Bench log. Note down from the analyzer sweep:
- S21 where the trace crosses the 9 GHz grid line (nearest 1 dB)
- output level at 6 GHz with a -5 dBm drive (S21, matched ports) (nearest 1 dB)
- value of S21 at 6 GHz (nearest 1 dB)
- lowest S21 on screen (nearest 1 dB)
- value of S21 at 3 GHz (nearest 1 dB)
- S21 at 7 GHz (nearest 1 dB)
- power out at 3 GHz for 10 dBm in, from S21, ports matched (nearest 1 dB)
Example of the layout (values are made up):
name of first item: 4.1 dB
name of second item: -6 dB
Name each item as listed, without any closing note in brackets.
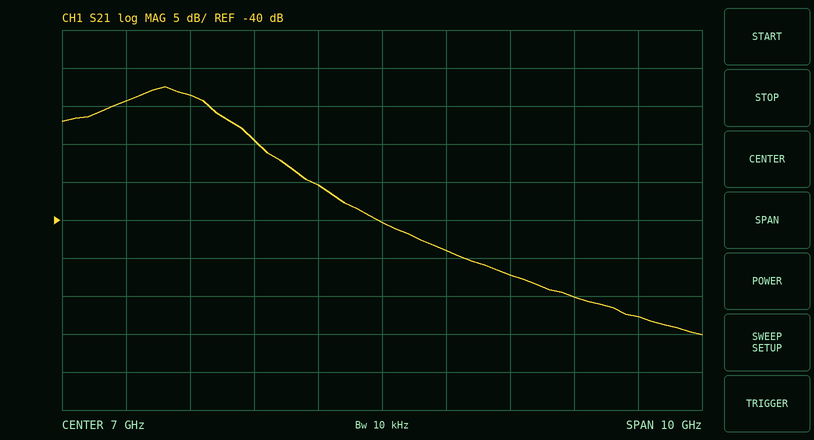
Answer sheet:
S21 where the trace crosses the 9 GHz grid line: -47 dB
output level at 6 GHz with a -5 dBm drive (S21, matched ports): -40 dBm
value of S21 at 6 GHz: -35 dB
lowest S21 on screen: -55 dB
value of S21 at 3 GHz: -24 dB
S21 at 7 GHz: -40 dB
power out at 3 GHz for 10 dBm in, from S21, ports matched: -14 dBm
